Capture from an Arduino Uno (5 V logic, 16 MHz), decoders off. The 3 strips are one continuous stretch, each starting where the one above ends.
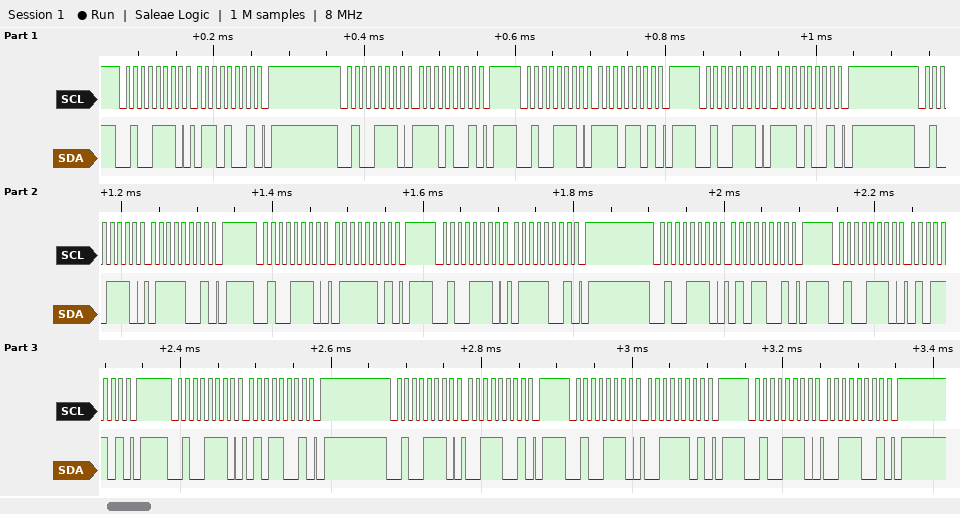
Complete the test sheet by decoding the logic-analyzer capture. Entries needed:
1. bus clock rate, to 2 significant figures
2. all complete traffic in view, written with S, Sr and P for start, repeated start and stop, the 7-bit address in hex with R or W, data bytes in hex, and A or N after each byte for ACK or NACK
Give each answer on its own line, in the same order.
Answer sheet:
100 kHz
S 27W A 69 A P S 27W A E9 A P S 27W A ED A P S 27W A E9 A P S 27W A 79 A P S 27W A 7D A P S 27W A 79 A P S 27W A 59 A P S 27W A 5D A P S 27W A 59 A P S 27W A 39 A P S 27W A 3D A P S 27W A 39 A P
